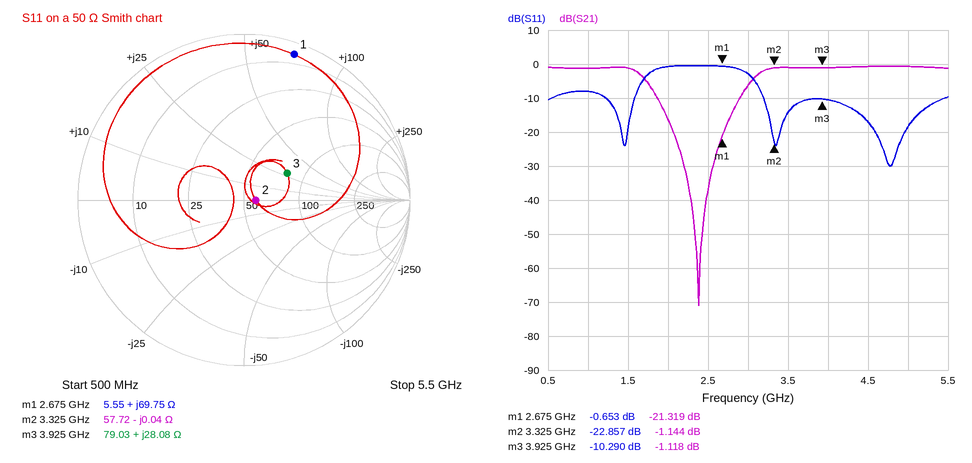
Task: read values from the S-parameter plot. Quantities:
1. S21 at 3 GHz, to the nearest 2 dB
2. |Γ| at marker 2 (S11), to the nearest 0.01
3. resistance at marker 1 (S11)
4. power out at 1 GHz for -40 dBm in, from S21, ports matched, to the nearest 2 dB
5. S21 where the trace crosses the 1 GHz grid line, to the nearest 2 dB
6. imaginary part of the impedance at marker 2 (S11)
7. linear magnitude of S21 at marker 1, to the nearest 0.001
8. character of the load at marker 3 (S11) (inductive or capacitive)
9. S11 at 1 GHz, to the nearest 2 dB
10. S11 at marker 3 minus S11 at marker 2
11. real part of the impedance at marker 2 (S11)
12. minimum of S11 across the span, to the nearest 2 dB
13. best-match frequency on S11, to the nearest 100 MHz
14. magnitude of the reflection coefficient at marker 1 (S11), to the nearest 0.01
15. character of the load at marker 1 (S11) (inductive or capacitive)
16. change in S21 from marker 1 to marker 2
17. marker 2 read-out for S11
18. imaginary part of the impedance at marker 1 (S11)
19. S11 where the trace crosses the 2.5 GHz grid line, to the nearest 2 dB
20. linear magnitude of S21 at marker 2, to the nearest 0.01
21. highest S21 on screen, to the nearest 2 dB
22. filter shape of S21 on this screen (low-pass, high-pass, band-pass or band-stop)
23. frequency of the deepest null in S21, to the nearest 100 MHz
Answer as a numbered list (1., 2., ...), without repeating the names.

1. -6 dB
2. 0.07
3. 5.55 Ω
4. -42 dBm
5. -2 dB
6. -0.04 Ω
7. 0.086
8. inductive
9. -8 dB
10. 12.567 dB
11. 57.72 Ω
12. -30 dB
13. 4.8 GHz
14. 0.93
15. inductive
16. 20.175 dB
17. -22.857 dB
18. +69.75 Ω
19. 0 dB
20. 0.88
21. 0 dB
22. band-stop
23. 2.4 GHz
